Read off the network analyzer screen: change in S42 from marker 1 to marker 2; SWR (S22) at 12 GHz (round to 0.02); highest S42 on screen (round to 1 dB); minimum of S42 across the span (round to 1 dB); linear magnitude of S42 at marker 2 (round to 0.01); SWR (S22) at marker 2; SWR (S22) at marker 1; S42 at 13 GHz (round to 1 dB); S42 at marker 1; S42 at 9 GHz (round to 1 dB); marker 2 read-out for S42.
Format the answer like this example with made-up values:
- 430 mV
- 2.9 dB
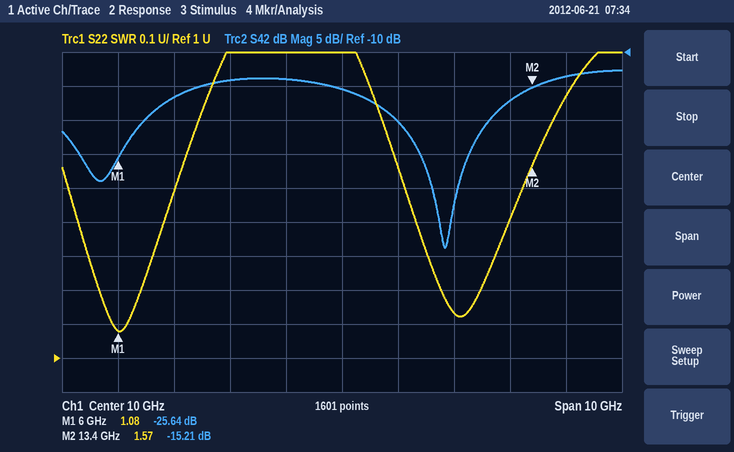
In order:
- 10.43 dB
- 1.14
- -13 dB
- -39 dB
- 0.17
- 1.57
- 1.08
- -17 dB
- -25.64 dB
- -14 dB
- -15.21 dB
